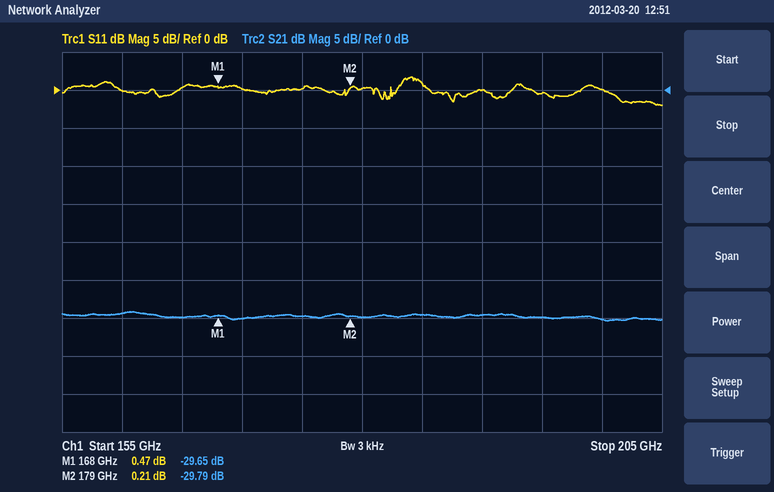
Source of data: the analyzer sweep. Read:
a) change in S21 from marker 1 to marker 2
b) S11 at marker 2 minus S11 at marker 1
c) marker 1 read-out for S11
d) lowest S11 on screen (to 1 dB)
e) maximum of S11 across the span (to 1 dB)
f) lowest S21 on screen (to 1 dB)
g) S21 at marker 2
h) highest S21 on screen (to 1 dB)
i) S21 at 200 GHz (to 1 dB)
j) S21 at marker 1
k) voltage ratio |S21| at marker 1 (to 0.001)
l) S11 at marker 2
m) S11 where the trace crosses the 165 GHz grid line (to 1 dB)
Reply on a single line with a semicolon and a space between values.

-0.14 dB; -0.26 dB; 0.47 dB; -2 dB; 2 dB; -30 dB; -29.79 dB; -29 dB; -30 dB; -29.65 dB; 0.033; 0.21 dB; 0 dB
